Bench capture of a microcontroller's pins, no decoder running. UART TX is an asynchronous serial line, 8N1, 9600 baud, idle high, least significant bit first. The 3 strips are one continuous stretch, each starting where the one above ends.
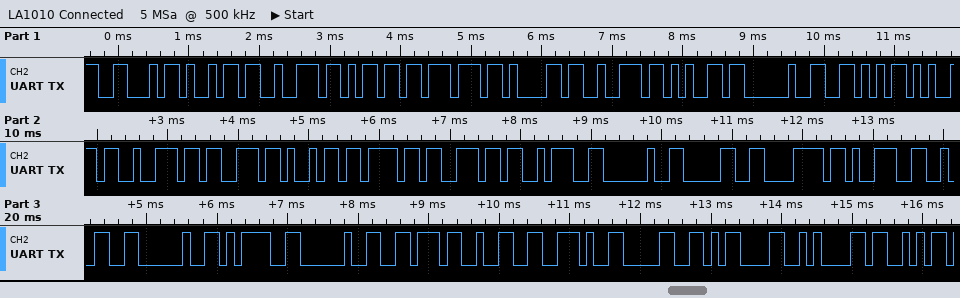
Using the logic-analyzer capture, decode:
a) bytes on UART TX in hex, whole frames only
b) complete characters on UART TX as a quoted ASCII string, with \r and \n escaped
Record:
46 69 72 6D 77 61 72 65 20 56 65 72 73 69 6F 6E 3A 20 30 78 39 32 20 3D 20 76 32 2E 30 0D 0A 53
"Firmware Version: 0x92 = v2.0\r\nS"
